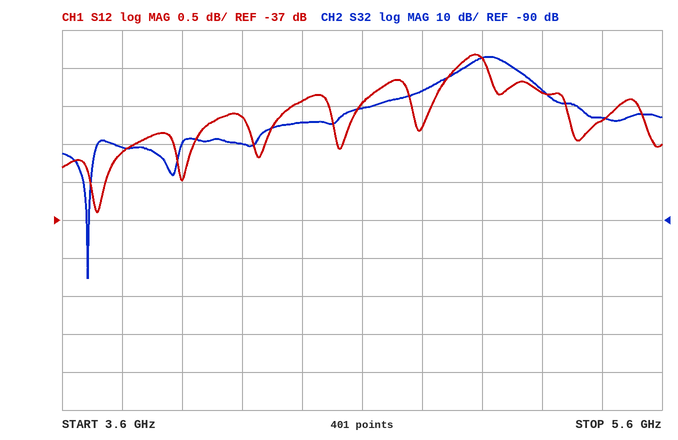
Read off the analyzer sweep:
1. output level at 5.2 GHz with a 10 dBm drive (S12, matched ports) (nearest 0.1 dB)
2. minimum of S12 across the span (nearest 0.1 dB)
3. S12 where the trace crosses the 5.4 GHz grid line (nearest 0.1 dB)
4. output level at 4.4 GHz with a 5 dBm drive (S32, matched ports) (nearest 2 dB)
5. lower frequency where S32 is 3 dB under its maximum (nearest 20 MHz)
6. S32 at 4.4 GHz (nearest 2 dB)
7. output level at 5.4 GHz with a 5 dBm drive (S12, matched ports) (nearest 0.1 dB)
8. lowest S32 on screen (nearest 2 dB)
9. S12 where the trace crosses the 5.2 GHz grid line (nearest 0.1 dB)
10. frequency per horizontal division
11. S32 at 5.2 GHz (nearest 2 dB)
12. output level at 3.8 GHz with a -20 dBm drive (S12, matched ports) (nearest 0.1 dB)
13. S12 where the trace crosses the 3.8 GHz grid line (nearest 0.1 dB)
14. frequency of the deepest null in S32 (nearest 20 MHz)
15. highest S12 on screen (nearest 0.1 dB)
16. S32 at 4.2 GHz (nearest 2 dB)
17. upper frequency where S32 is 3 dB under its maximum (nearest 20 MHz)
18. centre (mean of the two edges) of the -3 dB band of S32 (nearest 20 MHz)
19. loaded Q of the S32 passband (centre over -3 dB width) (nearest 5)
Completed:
-25.3 dBm
-36.9 dB
-35.7 dB
-60 dBm
4.94 GHz
-64 dB
-30.7 dBm
-106 dB
-35.3 dB
200 MHz
-56 dB
-56.1 dBm
-36.1 dB
3.68 GHz
-34.8 dB
-70 dB
5.10 GHz
5.02 GHz
30
